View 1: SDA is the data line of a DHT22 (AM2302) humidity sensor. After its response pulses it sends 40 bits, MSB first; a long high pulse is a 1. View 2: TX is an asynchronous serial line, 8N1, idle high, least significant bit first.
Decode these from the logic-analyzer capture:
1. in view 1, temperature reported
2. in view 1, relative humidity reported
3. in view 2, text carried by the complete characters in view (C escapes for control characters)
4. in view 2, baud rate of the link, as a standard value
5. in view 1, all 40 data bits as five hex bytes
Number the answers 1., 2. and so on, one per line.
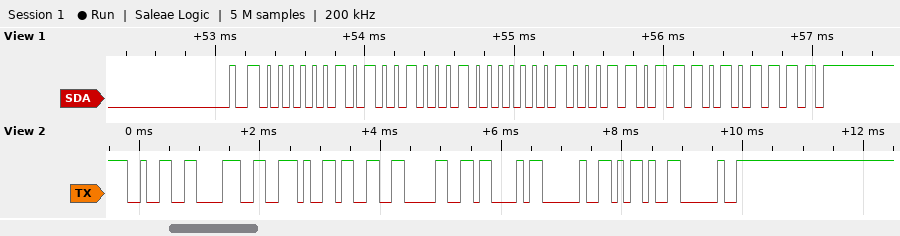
1. 28.3 °C
2. 65.7 %
3. "28.30C - "
4. 9600 baud
5. 02 91 01 1B AF
